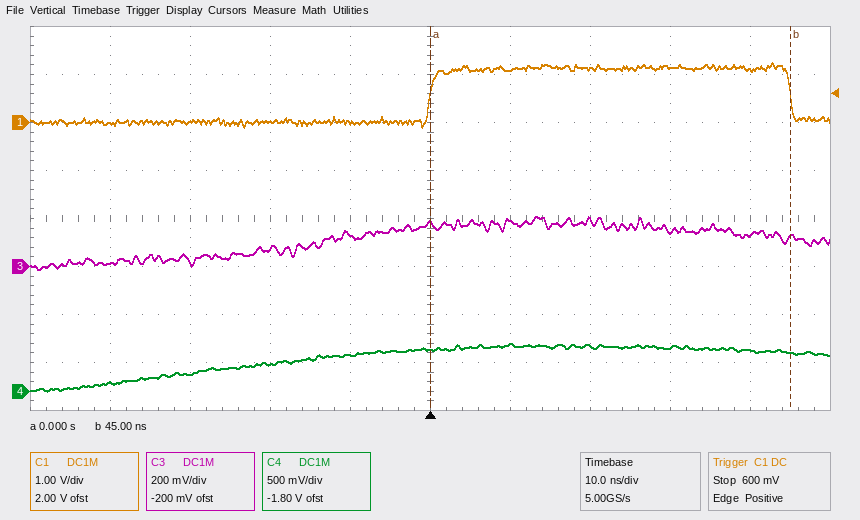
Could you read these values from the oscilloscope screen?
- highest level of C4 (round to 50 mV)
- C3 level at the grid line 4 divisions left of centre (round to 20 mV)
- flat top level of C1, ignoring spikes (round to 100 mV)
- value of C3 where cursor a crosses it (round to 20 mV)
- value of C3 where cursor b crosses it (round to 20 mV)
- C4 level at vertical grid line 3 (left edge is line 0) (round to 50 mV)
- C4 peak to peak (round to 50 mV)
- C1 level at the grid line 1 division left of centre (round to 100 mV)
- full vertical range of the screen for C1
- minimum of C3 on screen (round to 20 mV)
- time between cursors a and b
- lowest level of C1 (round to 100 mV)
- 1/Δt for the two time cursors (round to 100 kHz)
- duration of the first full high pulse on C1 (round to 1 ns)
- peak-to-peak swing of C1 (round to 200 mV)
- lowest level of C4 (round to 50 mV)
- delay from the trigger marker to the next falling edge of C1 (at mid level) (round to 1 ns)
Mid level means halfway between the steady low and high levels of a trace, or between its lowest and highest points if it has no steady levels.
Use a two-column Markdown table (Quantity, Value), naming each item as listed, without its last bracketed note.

| Quantity | Value |
|---|---|
| highest level of C4 | 500 mV |
| C3 level at the grid line 4 divisions left of centre | 20 mV |
| flat top level of C1, ignoring spikes | 1.1 V |
| value of C3 where cursor a crosses it | 180 mV |
| value of C3 where cursor b crosses it | 120 mV |
| C4 level at vertical grid line 3 (left edge is line 0) | 300 mV |
| C4 peak to peak | 500 mV |
| C1 level at the grid line 1 division left of centre | 0.0 V |
| full vertical range of the screen for C1 | 8 V |
| minimum of C3 on screen | -20 mV |
| time between cursors a and b | 45 ns |
| lowest level of C1 | -100 mV |
| 1/Δt for the two time cursors | 22.2 MHz |
| duration of the first full high pulse on C1 | 45 ns |
| peak-to-peak swing of C1 | 1.4 V |
| lowest level of C4 | 0 mV |
| delay from the trigger marker to the next falling edge of C1 (at mid level) | 45 ns |
